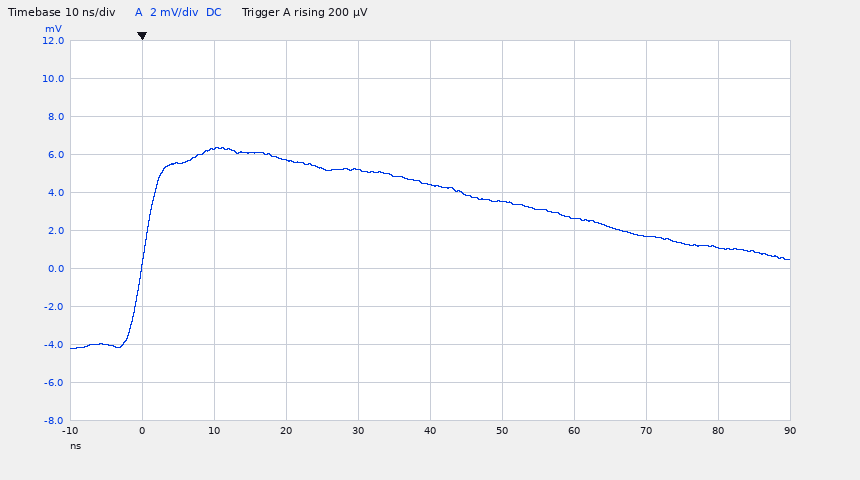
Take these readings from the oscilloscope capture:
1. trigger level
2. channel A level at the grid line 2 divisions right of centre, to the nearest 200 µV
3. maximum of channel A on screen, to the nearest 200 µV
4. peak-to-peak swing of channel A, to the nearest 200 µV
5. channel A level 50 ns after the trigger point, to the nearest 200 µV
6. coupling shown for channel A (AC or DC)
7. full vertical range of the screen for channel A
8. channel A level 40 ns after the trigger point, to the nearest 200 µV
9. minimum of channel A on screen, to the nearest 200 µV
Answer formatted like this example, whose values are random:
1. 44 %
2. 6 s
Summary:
1. 200 µV
2. 2.6 mV
3. 6.4 mV
4. 10.6 mV
5. 3.6 mV
6. DC
7. 20 mV
8. 4.4 mV
9. -4.2 mV
